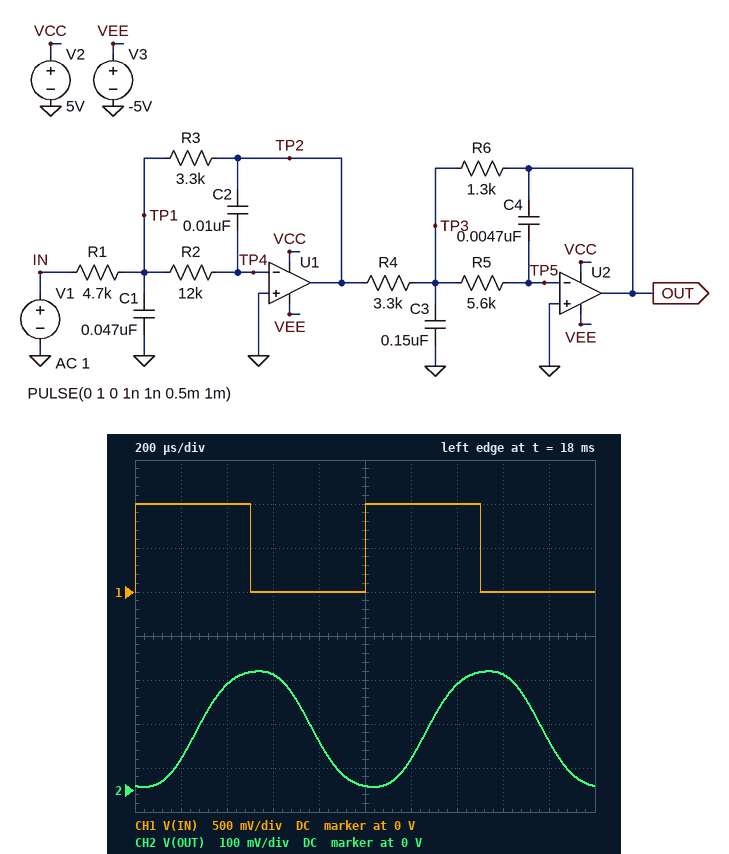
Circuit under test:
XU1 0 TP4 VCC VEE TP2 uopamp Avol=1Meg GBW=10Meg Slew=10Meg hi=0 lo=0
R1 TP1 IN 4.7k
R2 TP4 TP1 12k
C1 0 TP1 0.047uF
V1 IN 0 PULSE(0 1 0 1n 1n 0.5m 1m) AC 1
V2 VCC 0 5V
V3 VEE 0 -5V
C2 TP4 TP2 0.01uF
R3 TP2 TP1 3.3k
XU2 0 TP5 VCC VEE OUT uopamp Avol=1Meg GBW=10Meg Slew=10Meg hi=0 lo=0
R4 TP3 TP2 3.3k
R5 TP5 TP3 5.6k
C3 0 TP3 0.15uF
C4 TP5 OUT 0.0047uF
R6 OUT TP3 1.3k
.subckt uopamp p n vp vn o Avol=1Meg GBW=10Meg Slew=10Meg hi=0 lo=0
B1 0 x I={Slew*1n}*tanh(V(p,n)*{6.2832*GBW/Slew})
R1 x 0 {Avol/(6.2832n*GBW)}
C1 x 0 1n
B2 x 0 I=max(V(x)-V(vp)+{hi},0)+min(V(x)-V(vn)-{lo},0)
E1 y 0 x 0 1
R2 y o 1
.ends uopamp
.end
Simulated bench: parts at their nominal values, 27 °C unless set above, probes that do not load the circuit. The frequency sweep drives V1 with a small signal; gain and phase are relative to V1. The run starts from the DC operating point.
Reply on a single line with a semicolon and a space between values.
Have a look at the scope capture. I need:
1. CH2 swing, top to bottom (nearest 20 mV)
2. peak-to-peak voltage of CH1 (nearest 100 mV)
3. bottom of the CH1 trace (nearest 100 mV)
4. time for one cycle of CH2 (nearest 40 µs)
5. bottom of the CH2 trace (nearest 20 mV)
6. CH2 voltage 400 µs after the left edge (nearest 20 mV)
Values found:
260 mV; 1.0 V; 0 V; 1.00 ms; 0 V; 240 mV
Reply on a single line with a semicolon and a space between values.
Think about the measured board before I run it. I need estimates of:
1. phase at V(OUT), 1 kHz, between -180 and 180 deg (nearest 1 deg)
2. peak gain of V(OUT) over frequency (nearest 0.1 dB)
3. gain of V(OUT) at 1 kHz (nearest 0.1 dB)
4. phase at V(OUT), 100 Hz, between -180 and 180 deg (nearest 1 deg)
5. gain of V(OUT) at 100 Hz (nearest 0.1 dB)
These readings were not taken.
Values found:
-99 deg; -11.2 dB; -13.3 dB; -10 deg; -11.2 dB
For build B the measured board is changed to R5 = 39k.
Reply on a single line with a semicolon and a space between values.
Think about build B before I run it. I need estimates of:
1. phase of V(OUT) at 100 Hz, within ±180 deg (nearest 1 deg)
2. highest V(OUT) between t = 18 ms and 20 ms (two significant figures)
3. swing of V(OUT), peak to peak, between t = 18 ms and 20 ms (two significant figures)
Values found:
-18 deg; 210 mV; 140 mV
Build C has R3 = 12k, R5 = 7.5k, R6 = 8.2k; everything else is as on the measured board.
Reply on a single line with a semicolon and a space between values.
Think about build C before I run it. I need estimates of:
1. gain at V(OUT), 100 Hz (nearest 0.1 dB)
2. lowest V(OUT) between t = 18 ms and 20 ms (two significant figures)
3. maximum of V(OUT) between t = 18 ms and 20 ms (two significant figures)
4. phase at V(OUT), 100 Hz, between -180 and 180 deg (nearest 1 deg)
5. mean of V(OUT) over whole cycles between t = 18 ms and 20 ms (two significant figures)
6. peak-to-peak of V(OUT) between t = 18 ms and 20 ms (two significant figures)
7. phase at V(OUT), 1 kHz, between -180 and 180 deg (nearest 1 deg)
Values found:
15.9 dB; 2.3 V; 4.0 V; -25 deg; 3.2 V; 1.7 V; 119 deg
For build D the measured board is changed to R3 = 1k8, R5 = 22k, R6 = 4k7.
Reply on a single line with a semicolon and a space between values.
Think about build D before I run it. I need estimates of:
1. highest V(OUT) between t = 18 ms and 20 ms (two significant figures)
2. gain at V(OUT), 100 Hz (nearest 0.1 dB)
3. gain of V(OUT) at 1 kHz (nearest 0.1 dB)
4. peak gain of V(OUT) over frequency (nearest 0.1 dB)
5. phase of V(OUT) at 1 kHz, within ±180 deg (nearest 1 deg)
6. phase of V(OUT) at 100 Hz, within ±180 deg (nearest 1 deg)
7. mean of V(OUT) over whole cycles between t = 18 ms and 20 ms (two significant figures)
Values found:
380 mV; -5.2 dB; -15.7 dB; -4.4 dB; 160 deg; -17 deg; 270 mV
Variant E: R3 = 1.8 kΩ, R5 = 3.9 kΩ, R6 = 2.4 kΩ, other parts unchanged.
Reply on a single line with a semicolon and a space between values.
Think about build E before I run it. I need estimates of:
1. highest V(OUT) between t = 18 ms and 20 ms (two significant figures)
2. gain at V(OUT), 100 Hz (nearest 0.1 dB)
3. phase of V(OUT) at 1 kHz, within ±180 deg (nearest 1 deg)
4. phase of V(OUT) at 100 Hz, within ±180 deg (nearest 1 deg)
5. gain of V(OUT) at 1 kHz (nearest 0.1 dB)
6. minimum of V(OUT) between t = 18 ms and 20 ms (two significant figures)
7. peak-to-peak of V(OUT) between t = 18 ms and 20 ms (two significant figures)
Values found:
310 mV; -11.1 dB; -83 deg; -8 deg; -11.3 dB; -27 mV; 330 mV
